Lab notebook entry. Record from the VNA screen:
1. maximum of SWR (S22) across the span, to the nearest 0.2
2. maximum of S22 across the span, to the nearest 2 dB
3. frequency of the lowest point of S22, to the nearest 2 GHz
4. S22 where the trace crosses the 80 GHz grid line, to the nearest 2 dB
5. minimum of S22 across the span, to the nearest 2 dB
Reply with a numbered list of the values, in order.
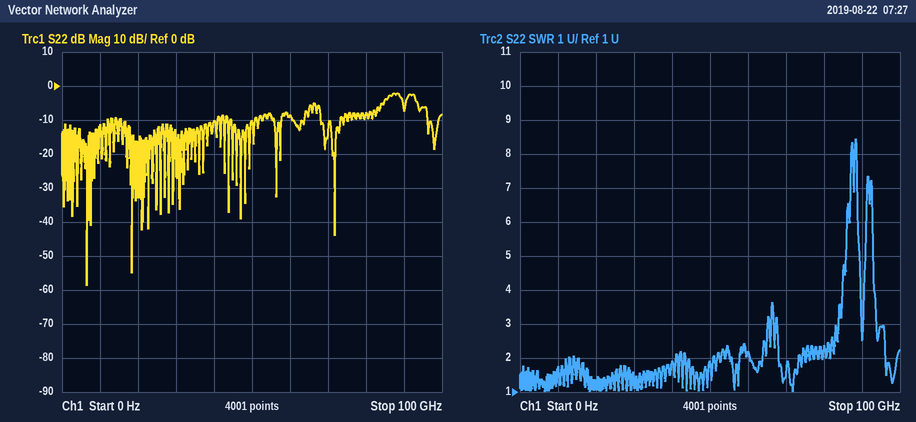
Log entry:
1. 8.4
2. -2 dB
3. 6 GHz
4. -8 dB
5. -58 dB
